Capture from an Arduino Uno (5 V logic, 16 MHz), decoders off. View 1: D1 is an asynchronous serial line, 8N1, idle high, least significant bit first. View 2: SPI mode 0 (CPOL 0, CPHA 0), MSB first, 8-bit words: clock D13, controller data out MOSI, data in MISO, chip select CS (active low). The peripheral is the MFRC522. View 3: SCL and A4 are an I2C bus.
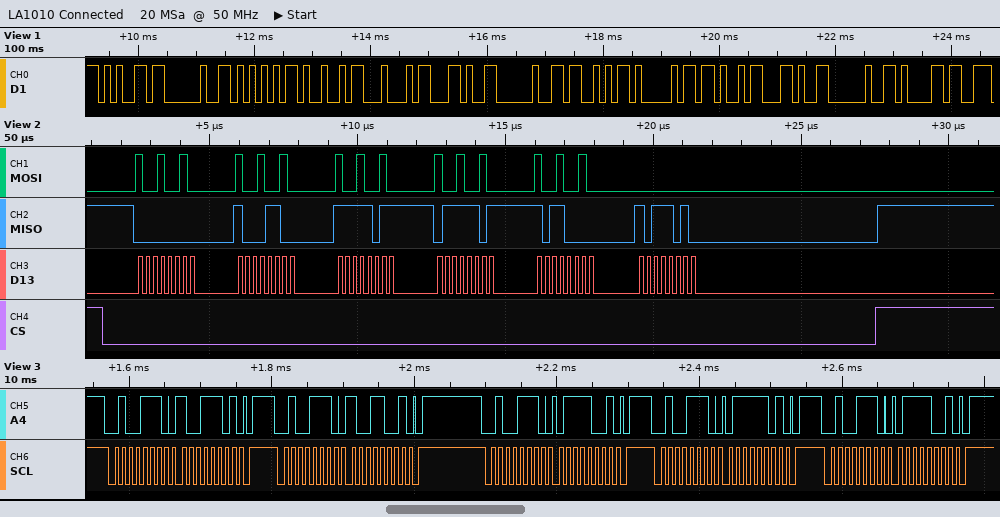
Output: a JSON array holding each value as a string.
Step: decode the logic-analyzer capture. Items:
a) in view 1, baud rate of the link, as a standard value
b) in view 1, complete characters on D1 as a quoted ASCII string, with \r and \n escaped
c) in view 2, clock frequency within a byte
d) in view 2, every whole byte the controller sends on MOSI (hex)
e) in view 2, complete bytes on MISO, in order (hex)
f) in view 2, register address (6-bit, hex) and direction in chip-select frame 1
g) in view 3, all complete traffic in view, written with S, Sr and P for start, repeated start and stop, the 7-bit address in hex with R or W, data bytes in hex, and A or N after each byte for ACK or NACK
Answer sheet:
["9600 baud", "\"e UID, SAK, a\"", "4 MHz", "92 92 92 92 92 00", "00 8C FB 7D B0 BA", "0x09 read", "S 27W A 9D A P S 27W A 99 A P S 27W A 79 A P S 27W A 7D A P S 27W A 79 A P"]
